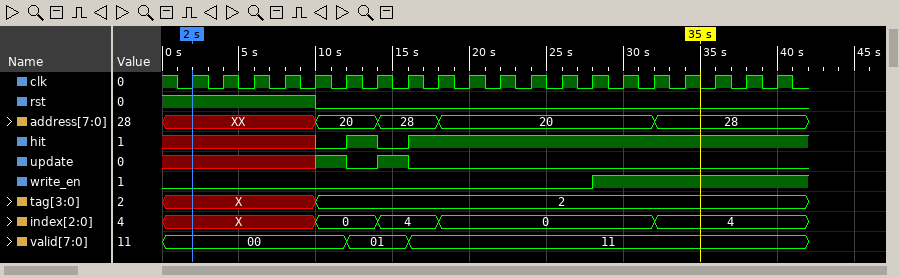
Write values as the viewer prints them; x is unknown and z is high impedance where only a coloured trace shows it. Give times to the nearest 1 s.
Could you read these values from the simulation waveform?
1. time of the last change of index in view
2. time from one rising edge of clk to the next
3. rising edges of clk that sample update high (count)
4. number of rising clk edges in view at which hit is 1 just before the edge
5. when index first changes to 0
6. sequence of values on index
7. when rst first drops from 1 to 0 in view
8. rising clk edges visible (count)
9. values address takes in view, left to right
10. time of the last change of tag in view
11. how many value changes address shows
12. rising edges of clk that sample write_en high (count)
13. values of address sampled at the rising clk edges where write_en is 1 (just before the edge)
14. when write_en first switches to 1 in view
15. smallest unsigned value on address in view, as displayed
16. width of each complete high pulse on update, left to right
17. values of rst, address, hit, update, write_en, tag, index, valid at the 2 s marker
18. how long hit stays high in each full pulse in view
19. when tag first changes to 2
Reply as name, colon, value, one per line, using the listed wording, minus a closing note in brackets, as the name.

time of the last change of index in view: 32 s
time from one rising edge of clk to the next: 2 s
rising edges of clk that sample update high: 2
number of rising clk edges in view at which hit is 1 just before the edge: 13
when index first changes to 0: 10 s
sequence of values on index: X, 0, 4, 0, 4
when rst first drops from 1 to 0 in view: 10 s
rising clk edges visible: 20
values address takes in view, left to right: XX, 20, 28, 20, 28
time of the last change of tag in view: 10 s
how many value changes address shows: 4
rising edges of clk that sample write_en high: 6
values of address sampled at the rising clk edges where write_en is 1: 20, 20, 28, 28, 28, 28
when write_en first switches to 1 in view: 28 s
smallest unsigned value on address in view, as displayed: 20
width of each complete high pulse on update, left to right: 2 s
values of rst, address, hit, update, write_en, tag, index, valid at the 2 s marker: rst=1, address=XX, hit=x, update=x, write_en=0, tag=X, index=X, valid=00
how long hit stays high in each full pulse in view: 2 s
when tag first changes to 2: 10 s
